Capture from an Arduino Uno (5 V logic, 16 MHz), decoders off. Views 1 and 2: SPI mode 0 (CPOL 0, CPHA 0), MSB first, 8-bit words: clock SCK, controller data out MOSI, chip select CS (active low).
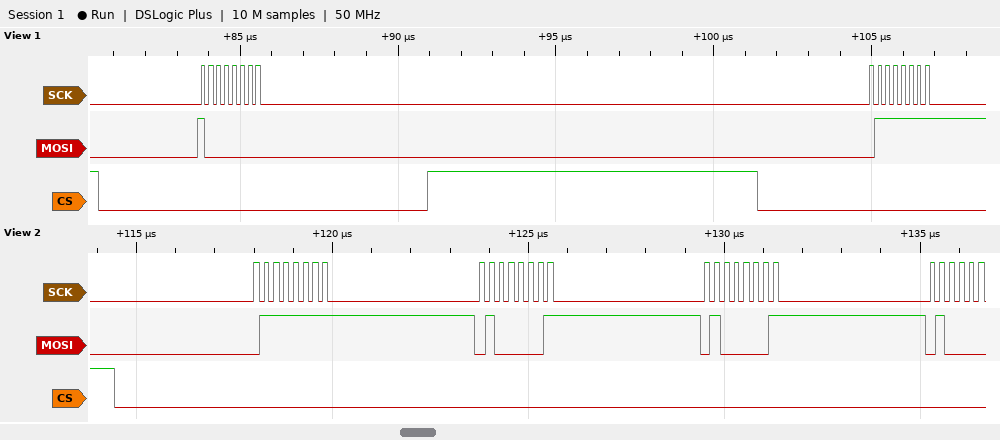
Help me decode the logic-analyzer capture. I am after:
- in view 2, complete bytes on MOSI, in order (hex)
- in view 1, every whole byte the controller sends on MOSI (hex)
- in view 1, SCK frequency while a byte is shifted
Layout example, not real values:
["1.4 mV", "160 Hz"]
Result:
["7F 41 41", "0x80 0x7F", "4 MHz"]
